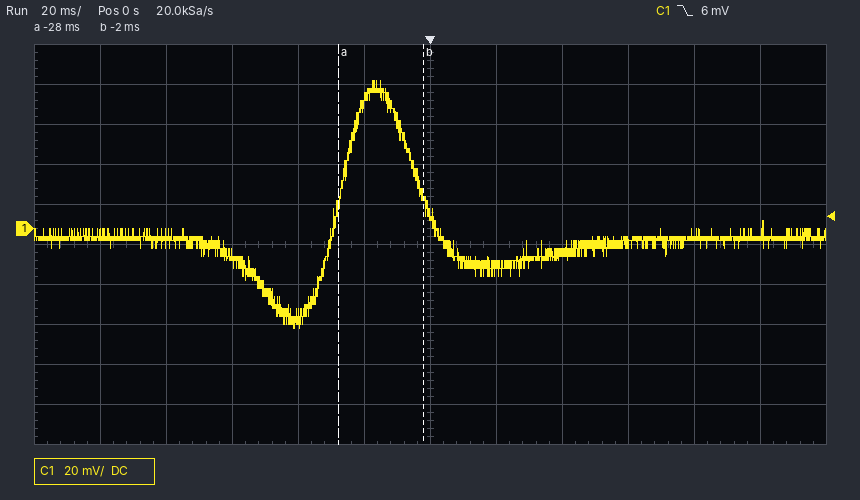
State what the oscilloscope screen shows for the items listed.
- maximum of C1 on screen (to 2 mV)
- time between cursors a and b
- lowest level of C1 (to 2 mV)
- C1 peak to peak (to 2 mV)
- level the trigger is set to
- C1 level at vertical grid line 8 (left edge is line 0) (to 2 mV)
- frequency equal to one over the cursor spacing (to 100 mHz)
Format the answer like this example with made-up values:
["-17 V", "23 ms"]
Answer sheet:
["74 mV", "26 ms", "-50 mV", "124 mV", "6 mV", "-12 mV", "38.5 Hz"]
